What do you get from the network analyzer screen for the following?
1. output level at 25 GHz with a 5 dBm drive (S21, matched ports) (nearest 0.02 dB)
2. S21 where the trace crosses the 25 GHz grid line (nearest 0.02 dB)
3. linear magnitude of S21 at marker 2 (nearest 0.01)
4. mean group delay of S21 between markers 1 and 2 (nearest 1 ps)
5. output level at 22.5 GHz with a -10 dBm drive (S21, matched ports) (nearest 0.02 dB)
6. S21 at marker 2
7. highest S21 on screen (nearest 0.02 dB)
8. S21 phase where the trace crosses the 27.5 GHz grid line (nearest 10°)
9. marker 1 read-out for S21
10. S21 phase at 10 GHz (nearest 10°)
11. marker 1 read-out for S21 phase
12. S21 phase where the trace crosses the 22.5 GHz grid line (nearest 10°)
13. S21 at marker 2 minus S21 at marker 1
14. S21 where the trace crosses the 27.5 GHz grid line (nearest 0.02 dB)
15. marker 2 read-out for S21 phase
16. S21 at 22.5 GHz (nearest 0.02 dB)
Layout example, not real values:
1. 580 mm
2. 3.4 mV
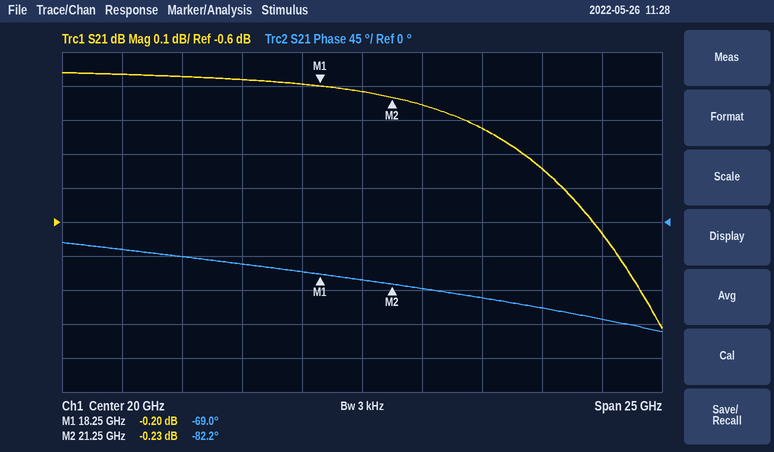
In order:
1. 4.68 dBm
2. -0.32 dB
3. 0.97
4. 12 ps
5. -10.26 dBm
6. -0.23 dB
7. -0.16 dB
8. -110°
9. -0.20 dB
10. -40°
11. -69.0°
12. -90°
13. -0.03 dB
14. -0.44 dB
15. -82.2°
16. -0.26 dB
